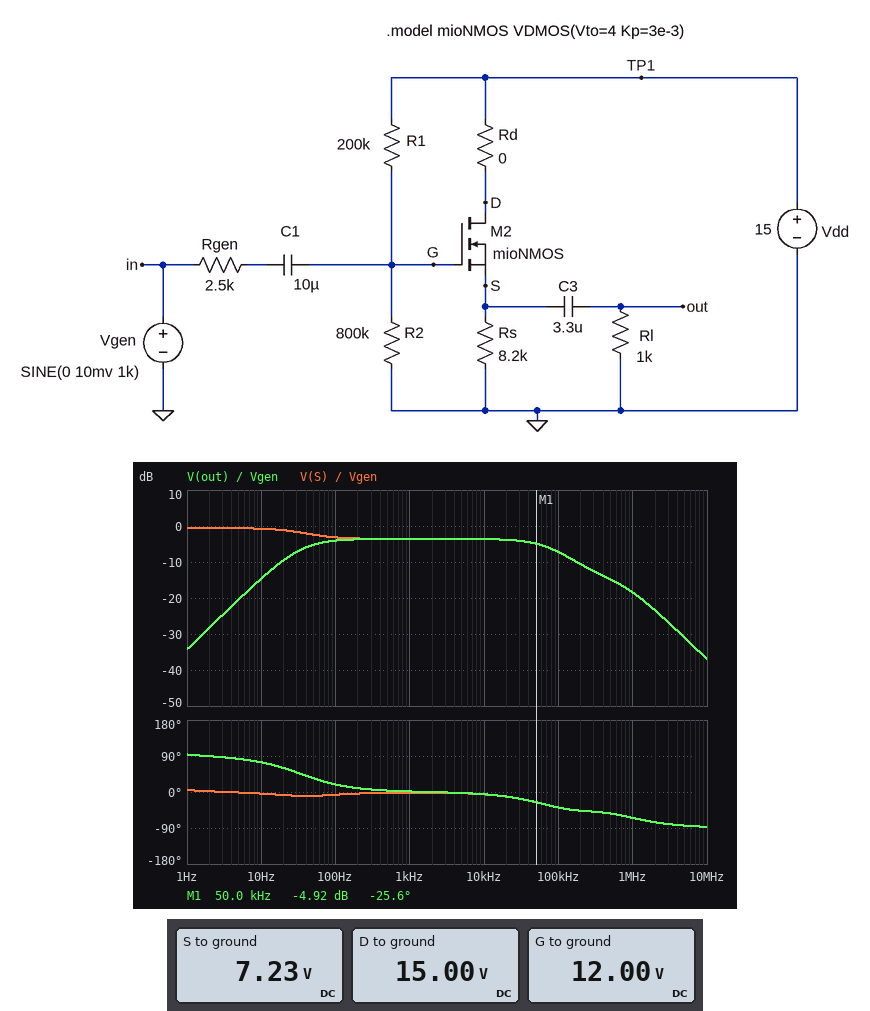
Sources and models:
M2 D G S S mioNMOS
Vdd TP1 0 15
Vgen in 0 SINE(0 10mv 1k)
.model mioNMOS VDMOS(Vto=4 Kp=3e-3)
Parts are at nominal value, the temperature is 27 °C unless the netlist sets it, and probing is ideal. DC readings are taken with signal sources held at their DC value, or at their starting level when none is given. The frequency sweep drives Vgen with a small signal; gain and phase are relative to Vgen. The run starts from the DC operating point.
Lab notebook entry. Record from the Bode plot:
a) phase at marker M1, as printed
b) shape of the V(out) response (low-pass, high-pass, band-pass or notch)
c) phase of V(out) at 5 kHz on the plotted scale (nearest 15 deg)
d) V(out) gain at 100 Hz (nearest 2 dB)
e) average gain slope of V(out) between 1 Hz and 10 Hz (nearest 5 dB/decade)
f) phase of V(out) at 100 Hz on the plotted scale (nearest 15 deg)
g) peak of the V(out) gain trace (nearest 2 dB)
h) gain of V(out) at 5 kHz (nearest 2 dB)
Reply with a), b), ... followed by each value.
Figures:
a) -25.6 deg
b) band-pass
c) 0 deg
d) -4 dB
e) 20 dB/decade
f) 15 deg
g) -4 dB
h) -4 dB
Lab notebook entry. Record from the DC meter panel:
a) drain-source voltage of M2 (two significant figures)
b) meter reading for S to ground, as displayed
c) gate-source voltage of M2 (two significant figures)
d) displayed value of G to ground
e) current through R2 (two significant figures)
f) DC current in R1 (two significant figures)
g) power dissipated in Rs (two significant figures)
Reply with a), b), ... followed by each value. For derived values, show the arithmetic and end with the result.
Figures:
a) 15 V - 7.23 V = 7.8 V
b) 7.23 V
c) 12 V - 7.23 V = 4.8 V
d) 12.00 V
e) (12 V) / 800 kΩ = 15 µA
f) (15 V - 12 V) / 200 kΩ = 15 µA
g) (7.23 V)^2 / 8.2 kΩ = 6.4 mW
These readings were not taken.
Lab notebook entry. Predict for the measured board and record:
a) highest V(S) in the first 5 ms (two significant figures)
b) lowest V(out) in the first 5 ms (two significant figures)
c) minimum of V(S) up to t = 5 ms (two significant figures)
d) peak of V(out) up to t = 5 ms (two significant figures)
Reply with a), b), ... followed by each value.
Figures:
a) 7.2 V
b) -6.8 mV
c) 7.2 V
d) 6.5 mV
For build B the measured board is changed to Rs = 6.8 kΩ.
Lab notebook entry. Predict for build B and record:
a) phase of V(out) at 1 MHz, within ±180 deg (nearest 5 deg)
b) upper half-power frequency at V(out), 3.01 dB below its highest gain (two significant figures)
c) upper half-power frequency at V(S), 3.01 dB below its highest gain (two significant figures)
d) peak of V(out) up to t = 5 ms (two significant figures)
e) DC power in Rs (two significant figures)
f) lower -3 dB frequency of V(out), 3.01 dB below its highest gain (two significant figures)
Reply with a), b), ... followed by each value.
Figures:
a) -65 deg
b) 88 kHz
c) 21 kHz
d) 6.7 mV
e) 7.5 mW
f) 35 Hz
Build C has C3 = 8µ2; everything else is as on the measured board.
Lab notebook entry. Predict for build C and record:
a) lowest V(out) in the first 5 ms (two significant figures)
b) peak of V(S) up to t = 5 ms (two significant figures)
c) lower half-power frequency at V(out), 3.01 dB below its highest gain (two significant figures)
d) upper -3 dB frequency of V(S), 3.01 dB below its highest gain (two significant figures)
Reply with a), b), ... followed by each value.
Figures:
a) -6.7 mV
b) 7.2 V
c) 14 Hz
d) 9.0 kHz
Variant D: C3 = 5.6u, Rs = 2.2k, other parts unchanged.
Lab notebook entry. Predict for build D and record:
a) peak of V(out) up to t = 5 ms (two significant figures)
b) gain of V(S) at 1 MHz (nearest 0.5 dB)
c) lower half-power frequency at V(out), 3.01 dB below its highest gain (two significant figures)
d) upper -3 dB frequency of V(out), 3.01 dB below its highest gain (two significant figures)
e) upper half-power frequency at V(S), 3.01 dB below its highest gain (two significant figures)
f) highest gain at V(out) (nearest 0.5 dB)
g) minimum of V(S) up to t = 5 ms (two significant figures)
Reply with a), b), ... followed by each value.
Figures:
a) 7.2 mV
b) -19.0 dB
c) 23 Hz
d) 100 kHz
e) 60 kHz
f) -2.5 dB
g) 6.6 V
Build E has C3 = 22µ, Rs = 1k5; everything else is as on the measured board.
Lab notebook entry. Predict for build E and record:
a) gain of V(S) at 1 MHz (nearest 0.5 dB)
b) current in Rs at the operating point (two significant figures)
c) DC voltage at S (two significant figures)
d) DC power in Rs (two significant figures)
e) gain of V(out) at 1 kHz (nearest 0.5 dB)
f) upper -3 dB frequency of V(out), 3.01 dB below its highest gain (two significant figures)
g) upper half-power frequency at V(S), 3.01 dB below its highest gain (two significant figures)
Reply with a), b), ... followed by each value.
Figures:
a) -19.0 dB
b) 4.2 mA
c) 6.3 V
d) 27 mW
e) -2.5 dB
f) 100 kHz
g) 69 kHz
